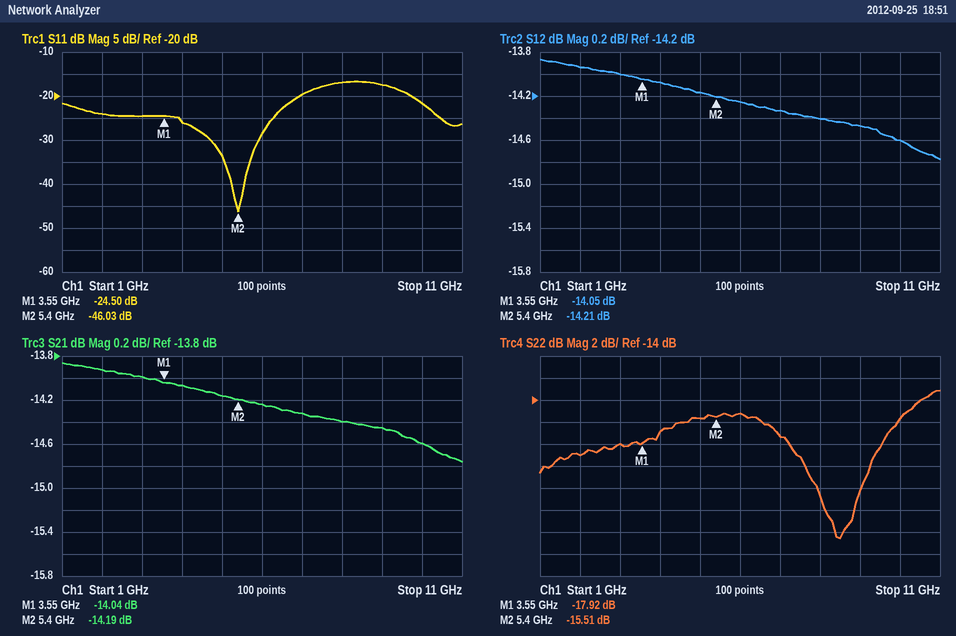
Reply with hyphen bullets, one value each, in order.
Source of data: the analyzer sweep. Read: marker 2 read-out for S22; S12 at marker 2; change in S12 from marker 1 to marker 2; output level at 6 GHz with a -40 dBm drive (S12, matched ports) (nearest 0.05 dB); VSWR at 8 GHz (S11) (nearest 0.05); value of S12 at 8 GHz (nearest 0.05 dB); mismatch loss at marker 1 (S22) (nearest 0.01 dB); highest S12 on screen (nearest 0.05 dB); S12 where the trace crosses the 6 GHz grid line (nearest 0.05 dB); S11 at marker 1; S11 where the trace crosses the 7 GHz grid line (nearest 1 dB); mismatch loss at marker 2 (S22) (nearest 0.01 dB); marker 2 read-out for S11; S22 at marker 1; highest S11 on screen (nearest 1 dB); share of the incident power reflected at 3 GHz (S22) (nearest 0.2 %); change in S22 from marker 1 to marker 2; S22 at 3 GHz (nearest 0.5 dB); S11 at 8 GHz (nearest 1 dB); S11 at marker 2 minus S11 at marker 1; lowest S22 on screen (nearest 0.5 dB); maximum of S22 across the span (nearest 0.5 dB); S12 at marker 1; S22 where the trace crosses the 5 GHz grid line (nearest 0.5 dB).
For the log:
- -15.51 dB
- -14.21 dB
- -0.16 dB
- -54.25 dBm
- 1.35
- -14.40 dB
- 0.07 dB
- -13.85 dB
- -14.25 dB
- -24.50 dB
- -20 dB
- 0.12 dB
- -46.03 dB
- -17.92 dB
- -17 dB
- 1.6 %
- 2.41 dB
- -18.0 dB
- -17 dB
- -21.53 dB
- -26.5 dB
- -13.0 dB
- -14.05 dB
- -15.5 dB
